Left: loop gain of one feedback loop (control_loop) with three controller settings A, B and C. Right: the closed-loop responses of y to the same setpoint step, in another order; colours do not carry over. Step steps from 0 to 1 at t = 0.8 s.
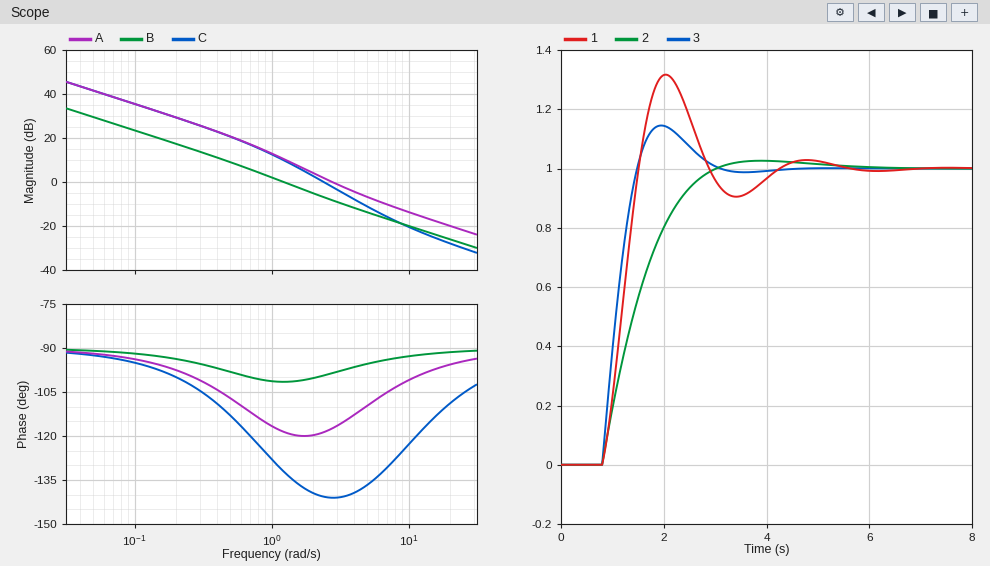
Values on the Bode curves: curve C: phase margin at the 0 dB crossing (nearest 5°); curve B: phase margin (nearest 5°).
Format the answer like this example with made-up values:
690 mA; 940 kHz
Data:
40°; 80°
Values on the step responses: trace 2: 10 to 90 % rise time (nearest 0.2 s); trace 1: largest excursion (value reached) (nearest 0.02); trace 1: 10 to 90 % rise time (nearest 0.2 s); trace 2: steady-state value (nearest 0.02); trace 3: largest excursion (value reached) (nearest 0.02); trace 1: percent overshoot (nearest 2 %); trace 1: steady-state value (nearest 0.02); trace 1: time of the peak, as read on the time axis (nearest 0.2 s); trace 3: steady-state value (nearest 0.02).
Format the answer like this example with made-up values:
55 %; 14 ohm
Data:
1.4 s; 1.32; 0.6 s; 1.00; 1.14; 32 %; 1.00; 2.0 s; 1.00
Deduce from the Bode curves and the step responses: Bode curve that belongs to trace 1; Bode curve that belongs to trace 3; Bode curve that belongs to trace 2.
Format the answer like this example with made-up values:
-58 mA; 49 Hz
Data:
C; A; B
